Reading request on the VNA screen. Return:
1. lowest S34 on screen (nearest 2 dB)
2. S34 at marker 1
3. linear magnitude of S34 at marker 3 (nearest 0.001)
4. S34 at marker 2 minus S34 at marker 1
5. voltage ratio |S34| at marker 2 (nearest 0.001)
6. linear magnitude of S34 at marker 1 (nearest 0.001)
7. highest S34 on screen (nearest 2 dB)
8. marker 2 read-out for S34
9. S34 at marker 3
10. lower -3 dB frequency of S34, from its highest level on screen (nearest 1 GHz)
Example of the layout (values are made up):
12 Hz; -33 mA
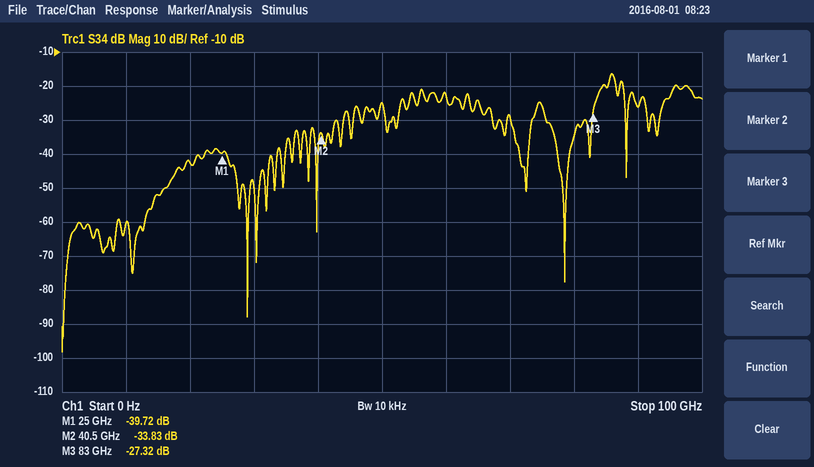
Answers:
-98 dB; -39.72 dB; 0.043; 5.89 dB; 0.020; 0.010; -16 dB; -33.83 dB; -27.32 dB; 85 GHz
